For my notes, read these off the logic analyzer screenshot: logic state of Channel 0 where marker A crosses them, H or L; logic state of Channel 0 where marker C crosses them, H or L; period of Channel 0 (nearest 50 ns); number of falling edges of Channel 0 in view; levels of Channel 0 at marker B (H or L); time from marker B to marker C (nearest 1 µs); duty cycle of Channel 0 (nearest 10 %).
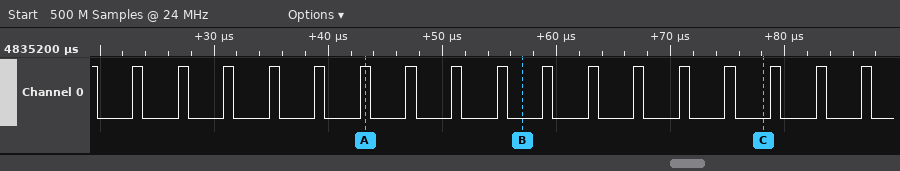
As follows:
Channel 0=H
Channel 0=L
4000 ns
18
Channel 0=L
21 µs
20 %
